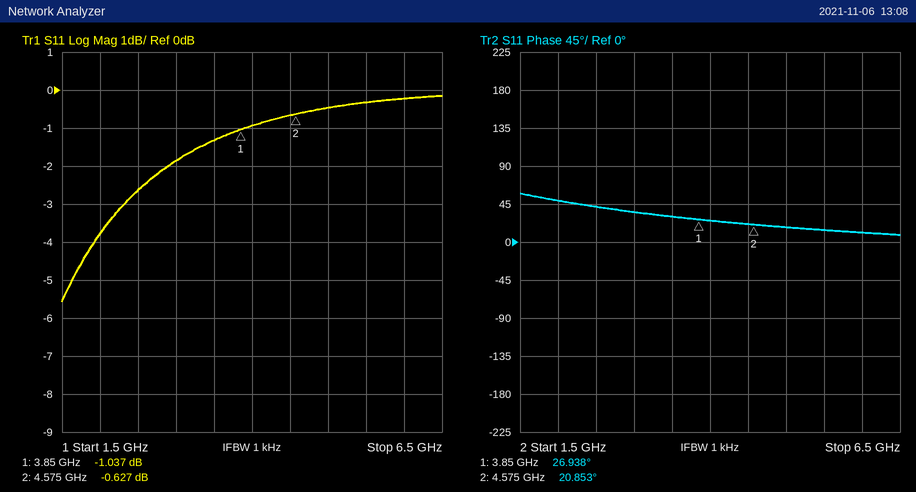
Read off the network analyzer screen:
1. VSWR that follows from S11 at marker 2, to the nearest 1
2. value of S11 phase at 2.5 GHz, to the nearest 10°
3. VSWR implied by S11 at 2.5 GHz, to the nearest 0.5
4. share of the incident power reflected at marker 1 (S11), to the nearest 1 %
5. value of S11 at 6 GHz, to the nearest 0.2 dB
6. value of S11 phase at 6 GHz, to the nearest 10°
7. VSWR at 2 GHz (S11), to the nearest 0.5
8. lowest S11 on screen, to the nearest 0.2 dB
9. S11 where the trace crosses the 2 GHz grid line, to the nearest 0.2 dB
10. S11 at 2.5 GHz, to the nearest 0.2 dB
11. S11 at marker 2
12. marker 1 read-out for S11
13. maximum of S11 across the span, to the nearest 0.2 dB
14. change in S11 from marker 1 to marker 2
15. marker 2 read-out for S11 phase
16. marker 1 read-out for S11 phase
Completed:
28
40°
6.5
79 %
-0.2 dB
10°
4.5
-5.6 dB
-3.8 dB
-2.6 dB
-0.627 dB
-1.037 dB
-0.2 dB
0.410 dB
20.853°
26.938°
